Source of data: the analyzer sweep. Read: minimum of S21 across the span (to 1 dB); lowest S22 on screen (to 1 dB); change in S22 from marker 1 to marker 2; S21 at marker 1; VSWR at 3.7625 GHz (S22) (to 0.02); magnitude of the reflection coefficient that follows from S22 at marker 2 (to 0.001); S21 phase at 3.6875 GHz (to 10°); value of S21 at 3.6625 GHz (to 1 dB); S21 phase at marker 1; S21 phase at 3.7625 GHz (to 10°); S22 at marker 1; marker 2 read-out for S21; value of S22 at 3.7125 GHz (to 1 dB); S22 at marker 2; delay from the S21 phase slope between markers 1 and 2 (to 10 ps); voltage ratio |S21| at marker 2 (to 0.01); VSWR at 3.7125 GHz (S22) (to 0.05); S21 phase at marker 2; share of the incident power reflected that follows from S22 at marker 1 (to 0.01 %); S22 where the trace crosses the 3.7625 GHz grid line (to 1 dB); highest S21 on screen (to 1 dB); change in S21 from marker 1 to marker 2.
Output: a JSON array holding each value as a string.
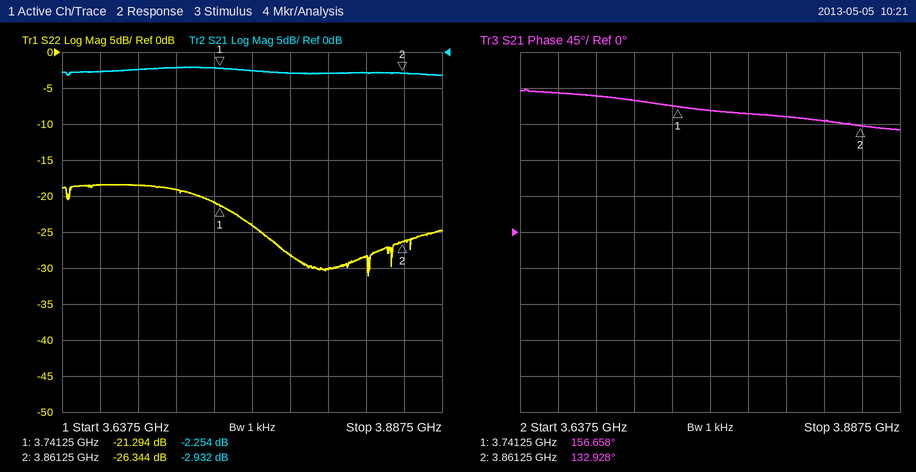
["-3 dB", "-31 dB", "-5.050 dB", "-2.254 dB", "1.14", "0.048", "170°", "-3 dB", "156.658°", "150°", "-21.294 dB", "-2.932 dB", "-19 dB", "-26.344 dB", "550 ps", "0.71", "1.25", "132.928°", "0.74 %", "-24 dB", "-2 dB", "-0.678 dB"]
